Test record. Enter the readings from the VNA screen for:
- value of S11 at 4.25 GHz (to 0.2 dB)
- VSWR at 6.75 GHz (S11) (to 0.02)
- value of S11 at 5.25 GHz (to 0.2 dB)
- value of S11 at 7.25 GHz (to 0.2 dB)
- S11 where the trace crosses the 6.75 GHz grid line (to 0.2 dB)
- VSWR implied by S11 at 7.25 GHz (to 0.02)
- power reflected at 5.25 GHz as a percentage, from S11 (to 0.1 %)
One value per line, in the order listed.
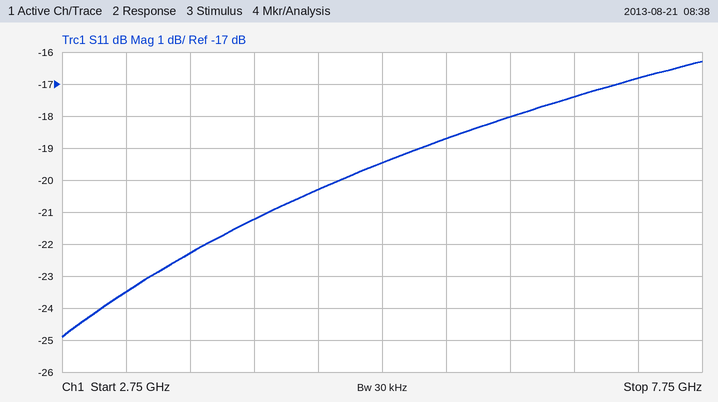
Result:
-21.2 dB
1.32
-19.4 dB
-16.8 dB
-17.4 dB
1.34
1.1 %
